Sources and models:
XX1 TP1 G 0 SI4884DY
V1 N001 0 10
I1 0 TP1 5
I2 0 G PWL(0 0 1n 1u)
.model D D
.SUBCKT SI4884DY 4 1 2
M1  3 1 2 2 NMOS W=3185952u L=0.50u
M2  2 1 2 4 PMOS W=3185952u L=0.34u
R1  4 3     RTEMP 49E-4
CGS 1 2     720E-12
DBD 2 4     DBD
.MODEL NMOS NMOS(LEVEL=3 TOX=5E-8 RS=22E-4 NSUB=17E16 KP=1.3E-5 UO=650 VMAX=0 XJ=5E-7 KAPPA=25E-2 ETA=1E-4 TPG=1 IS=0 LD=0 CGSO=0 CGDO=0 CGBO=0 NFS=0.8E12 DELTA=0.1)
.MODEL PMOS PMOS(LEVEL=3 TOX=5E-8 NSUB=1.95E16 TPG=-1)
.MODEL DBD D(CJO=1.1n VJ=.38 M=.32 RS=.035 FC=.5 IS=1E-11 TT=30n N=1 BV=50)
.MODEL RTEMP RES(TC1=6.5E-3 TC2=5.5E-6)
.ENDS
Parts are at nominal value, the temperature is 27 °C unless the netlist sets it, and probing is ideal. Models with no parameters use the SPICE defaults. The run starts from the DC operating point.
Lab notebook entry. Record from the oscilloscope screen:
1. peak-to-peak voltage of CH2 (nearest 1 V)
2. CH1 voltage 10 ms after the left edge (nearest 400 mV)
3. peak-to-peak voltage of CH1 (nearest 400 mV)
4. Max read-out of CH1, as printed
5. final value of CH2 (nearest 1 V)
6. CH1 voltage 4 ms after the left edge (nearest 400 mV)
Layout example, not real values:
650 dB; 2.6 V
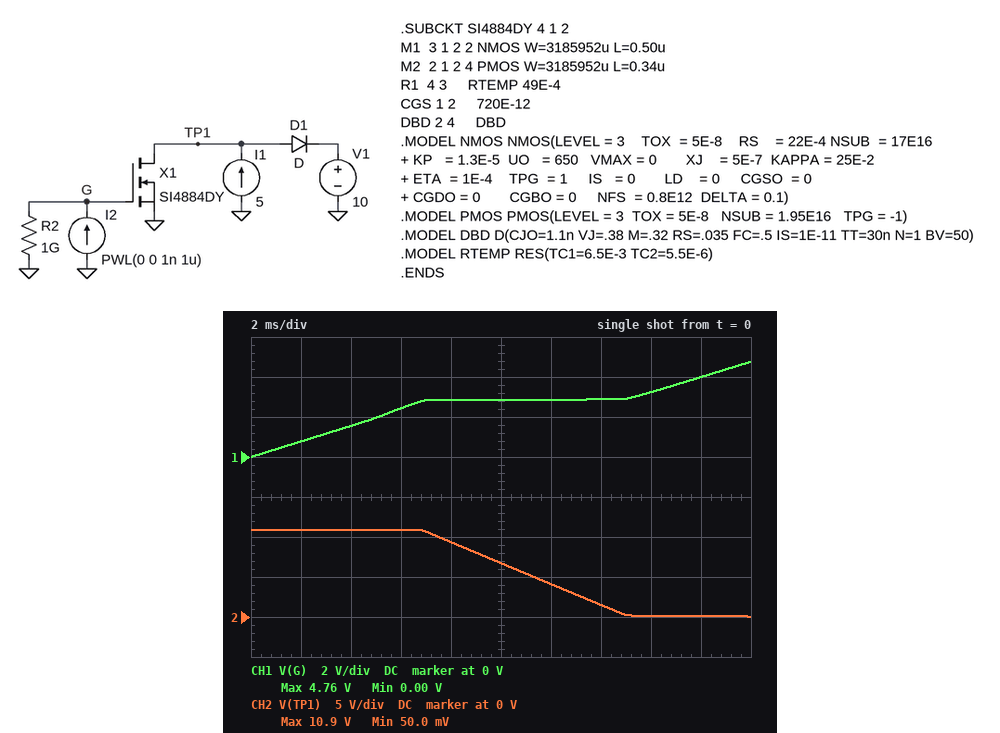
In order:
11 V; 2.8 V; 4.8 V; 4.76 V; 0 V; 1.6 V
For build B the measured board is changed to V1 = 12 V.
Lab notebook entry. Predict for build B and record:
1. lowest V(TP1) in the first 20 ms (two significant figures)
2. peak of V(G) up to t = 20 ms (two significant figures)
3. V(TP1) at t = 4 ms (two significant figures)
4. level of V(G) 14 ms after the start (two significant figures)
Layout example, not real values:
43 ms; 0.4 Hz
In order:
71 mV; 4.2 V; 13 V; 2.9 V
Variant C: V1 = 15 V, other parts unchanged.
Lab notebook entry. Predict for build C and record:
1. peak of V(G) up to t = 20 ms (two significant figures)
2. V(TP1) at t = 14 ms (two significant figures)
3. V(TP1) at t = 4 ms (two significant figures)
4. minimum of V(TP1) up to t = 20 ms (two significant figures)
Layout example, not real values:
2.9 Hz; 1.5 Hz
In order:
3.3 V; 6.4 V; 16 V; 110 mV
